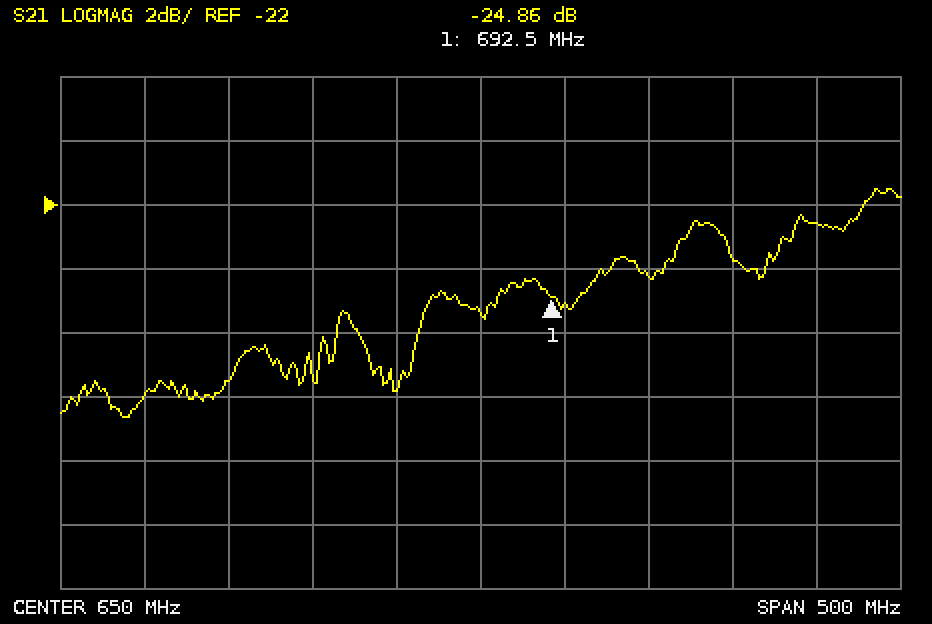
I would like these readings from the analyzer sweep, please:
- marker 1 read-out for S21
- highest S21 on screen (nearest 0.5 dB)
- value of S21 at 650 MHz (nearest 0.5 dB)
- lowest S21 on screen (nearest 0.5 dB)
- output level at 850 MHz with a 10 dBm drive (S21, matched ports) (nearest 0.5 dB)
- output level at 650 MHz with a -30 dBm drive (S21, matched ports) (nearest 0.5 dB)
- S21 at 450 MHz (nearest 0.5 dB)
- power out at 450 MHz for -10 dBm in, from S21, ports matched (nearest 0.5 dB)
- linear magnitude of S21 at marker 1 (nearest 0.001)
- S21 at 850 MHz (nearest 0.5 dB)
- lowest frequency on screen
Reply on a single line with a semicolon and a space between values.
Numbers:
-24.86 dB; -21.5 dB; -25.5 dB; -28.5 dB; -12.5 dBm; -55.5 dBm; -28.0 dB; -38.0 dBm; 0.057; -22.5 dB; 400 MHz
